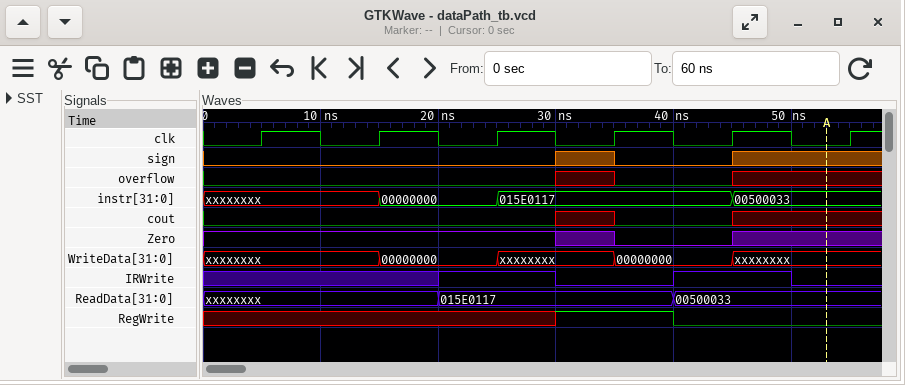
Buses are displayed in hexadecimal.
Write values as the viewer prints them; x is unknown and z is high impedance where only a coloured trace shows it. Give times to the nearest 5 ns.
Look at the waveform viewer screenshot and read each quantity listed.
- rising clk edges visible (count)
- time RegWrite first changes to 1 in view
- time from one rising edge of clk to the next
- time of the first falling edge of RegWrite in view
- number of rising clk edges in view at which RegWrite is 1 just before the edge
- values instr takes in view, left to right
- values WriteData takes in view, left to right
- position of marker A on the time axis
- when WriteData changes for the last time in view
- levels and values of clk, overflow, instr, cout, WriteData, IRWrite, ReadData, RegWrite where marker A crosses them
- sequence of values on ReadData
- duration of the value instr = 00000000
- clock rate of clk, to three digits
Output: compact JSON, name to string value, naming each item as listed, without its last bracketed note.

{"rising clk edges visible": "6", "time RegWrite first changes to 1 in view": "30 ns", "time from one rising edge of clk to the next": "10 ns", "time of the first falling edge of RegWrite in view": "40 ns", "number of rising clk edges in view at which RegWrite is 1 just before the edge": "1", "values instr takes in view, left to right": "xxxxxxxx, 00000000, 015E0117, 00500033", "values WriteData takes in view, left to right": "xxxxxxxx, 00000000, xxxxxxxx, 00000000, xxxxxxxx", "position of marker A on the time axis": "55 ns", "when WriteData changes for the last time in view": "45 ns", "levels and values of clk, overflow, instr, cout, WriteData, IRWrite, ReadData, RegWrite where marker A crosses them": "clk=0, overflow=x, instr=00500033, cout=x, WriteData=xxxxxxxx, IRWrite=0, ReadData=00500033, RegWrite=0", "sequence of values on ReadData": "xxxxxxxx, 015E0117, 00500033", "duration of the value instr = 00000000": "10 ns", "clock rate of clk, to three digits": "100 MHz"}
